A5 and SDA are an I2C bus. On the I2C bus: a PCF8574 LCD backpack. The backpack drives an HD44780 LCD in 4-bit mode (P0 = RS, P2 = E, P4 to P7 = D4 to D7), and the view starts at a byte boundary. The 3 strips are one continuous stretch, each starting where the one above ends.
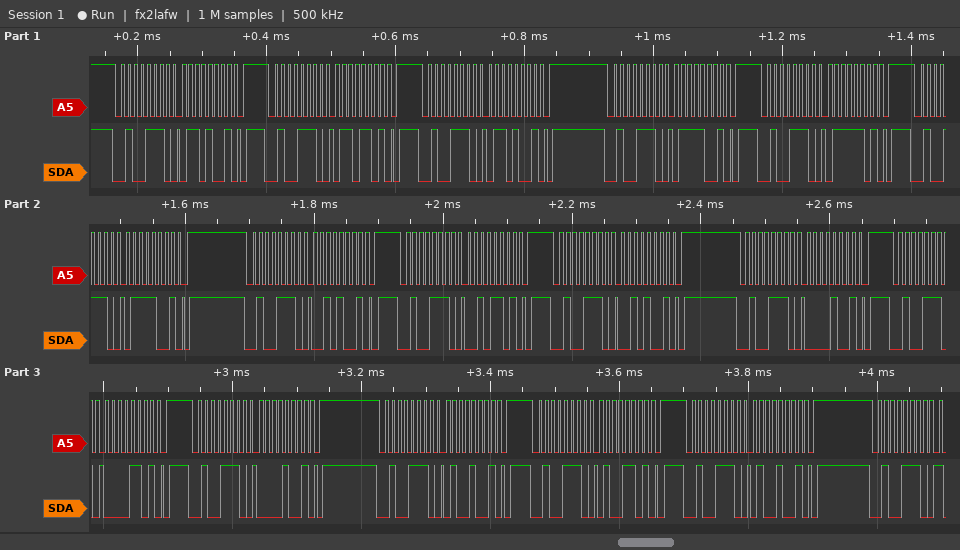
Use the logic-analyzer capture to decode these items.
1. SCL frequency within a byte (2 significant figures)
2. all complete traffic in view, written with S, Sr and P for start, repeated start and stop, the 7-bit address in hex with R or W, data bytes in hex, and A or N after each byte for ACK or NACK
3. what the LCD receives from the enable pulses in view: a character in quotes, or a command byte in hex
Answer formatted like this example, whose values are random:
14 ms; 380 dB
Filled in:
100 kHz; S 27W A 69 A P S 27W A 6D A P S 27W A 69 A P S 27W A 79 A P S 27W A 7D A P S 27W A 79 A P S 27W A 29 A P S 27W A 2D A P S 27W A 29 A P S 27W A 09 A P S 27W A 0D A P S 27W A 09 A P S 27W A 49 A P S 27W A 4D A P S 27W A 49 A P S 27W A; 'g' ' '
